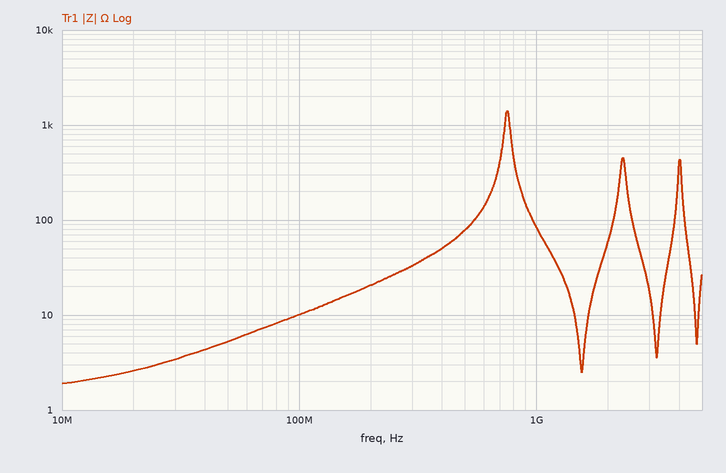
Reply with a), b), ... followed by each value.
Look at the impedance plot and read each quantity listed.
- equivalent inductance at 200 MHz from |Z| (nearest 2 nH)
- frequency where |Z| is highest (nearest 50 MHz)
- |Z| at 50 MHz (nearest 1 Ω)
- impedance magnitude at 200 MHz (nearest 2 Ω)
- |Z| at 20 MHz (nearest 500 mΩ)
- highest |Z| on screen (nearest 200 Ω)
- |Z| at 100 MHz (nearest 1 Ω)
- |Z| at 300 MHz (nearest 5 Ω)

a) 16 nH
b) 750 MHz
c) 5 Ω
d) 20 Ω
e) 2.5 Ω
f) 1.4 kΩ
g) 10 Ω
h) 35 Ω
